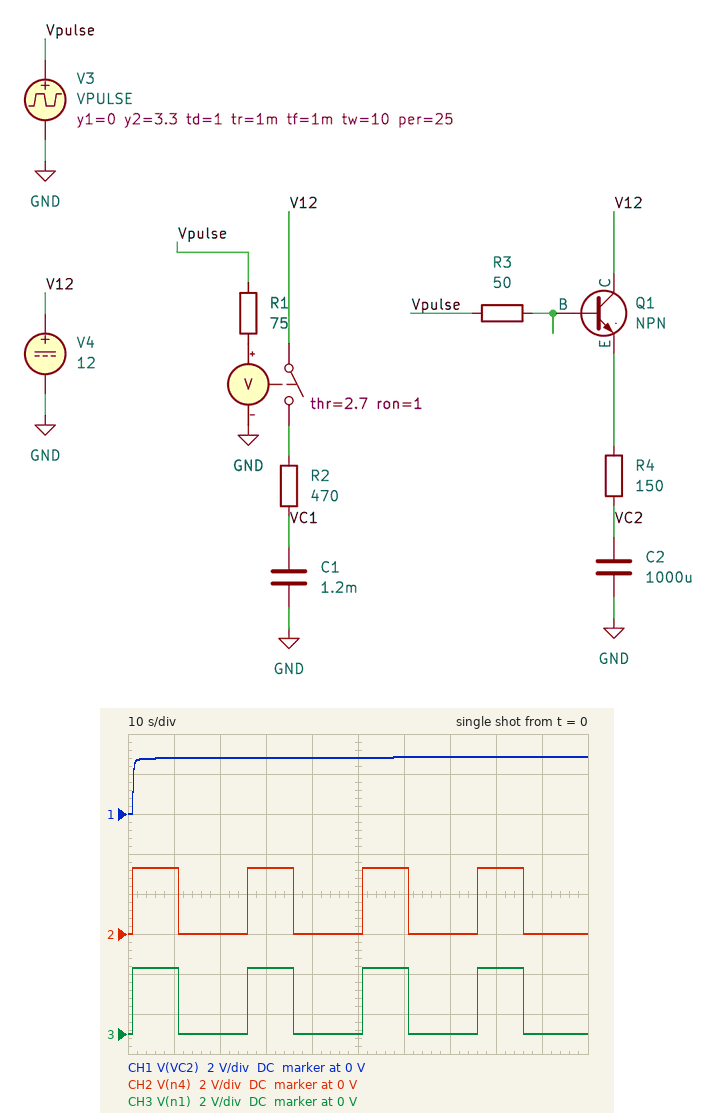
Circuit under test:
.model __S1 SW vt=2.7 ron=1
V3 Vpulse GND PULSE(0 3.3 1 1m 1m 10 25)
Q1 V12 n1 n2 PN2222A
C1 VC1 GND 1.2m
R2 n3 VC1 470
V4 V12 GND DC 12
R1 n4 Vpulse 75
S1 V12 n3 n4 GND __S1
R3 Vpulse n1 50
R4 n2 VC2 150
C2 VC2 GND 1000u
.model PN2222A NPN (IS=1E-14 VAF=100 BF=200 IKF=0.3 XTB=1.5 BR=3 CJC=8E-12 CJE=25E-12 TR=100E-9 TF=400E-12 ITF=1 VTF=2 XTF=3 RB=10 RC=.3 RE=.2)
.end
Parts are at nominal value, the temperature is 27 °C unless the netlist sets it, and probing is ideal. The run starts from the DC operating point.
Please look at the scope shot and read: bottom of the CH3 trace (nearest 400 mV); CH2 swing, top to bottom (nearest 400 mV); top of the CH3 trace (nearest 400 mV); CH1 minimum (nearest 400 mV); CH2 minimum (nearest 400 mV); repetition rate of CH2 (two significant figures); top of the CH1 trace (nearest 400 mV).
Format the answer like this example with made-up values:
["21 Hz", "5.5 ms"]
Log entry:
["0 V", "3.2 V", "3.2 V", "0 V", "0 V", "40 mHz", "2.8 V"]
